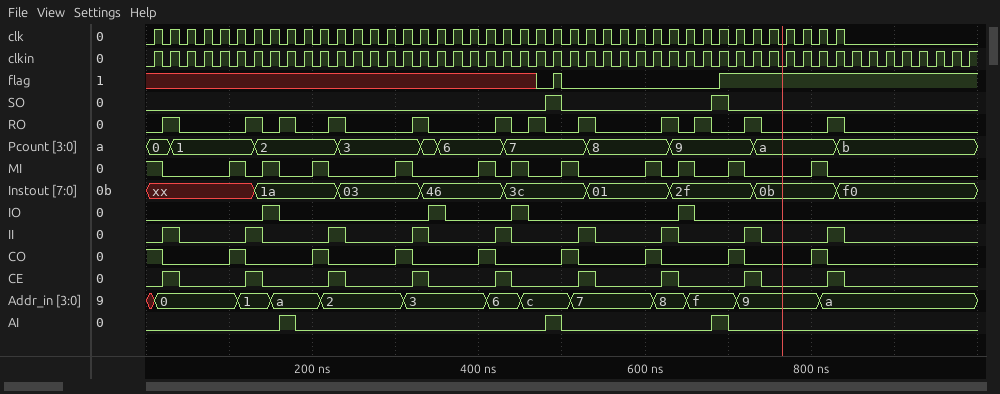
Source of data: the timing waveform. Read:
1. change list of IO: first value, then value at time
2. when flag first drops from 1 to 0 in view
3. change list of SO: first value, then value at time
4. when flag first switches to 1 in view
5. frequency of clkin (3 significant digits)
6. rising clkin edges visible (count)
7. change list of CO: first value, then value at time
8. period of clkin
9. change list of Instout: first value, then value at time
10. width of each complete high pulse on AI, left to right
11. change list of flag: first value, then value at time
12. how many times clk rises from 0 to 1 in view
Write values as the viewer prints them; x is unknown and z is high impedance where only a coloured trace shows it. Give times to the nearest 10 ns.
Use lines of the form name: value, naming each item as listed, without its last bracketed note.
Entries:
change list of IO: first value, then value at time: 0, 1 at 140 ns, 0 at 160 ns, 1 at 340 ns, 0 at 360 ns, 1 at 440 ns, 0 at 460 ns, 1 at 640 ns, 0 at 660 ns
when flag first drops from 1 to 0 in view: 500 ns
change list of SO: first value, then value at time: 0, 1 at 480 ns, 0 at 500 ns, 1 at 680 ns, 0 at 700 ns
when flag first switches to 1 in view: 490 ns
frequency of clkin: 50.0 MHz
rising clkin edges visible: 50
change list of CO: first value, then value at time: 1, 0 at 20 ns, 1 at 100 ns, 0 at 120 ns, 1 at 200 ns, 0 at 220 ns, 1 at 300 ns, 0 at 320 ns, 1 at 400 ns, 0 at 420 ns, 1 at 500 ns, 0 at 520 ns, 1 at 600 ns, 0 at 620 ns, 1 at 700 ns, 0 at 720 ns, 1 at 800 ns, 0 at 820 ns
period of clkin: 20 ns
change list of Instout: first value, then value at time: xx, 1a at 130 ns, 03 at 230 ns, 46 at 330 ns, 3c at 430 ns, 01 at 530 ns, 2f at 630 ns, 0b at 730 ns, f0 at 830 ns
width of each complete high pulse on AI, left to right: 20 ns, 20 ns, 20 ns
change list of flag: first value, then value at time: x, 0 at 470 ns, 1 at 490 ns, 0 at 500 ns, 1 at 690 ns
how many times clk rises from 0 to 1 in view: 42
